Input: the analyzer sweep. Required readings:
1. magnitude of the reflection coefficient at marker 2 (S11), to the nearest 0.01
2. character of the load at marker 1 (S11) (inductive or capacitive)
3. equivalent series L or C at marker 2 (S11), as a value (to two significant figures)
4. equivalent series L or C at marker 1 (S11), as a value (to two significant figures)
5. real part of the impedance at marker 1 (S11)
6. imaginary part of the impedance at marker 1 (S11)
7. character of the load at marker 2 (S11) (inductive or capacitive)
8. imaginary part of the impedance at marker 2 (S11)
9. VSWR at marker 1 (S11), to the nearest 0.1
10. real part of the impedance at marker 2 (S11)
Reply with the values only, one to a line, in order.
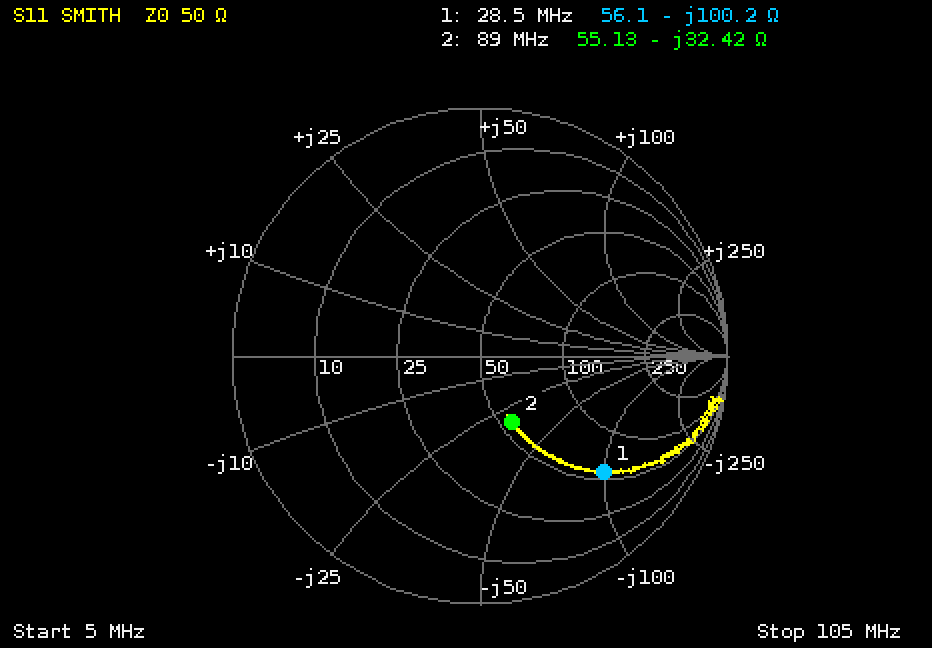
0.30
capacitive
55 pF
56 pF
56.1 Ω
-100.2 Ω
capacitive
-32.42 Ω
5.4
55.13 Ω
